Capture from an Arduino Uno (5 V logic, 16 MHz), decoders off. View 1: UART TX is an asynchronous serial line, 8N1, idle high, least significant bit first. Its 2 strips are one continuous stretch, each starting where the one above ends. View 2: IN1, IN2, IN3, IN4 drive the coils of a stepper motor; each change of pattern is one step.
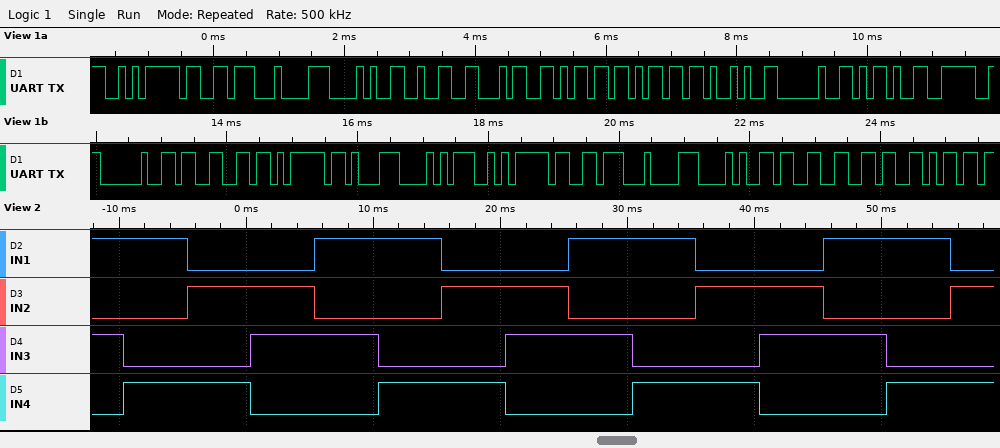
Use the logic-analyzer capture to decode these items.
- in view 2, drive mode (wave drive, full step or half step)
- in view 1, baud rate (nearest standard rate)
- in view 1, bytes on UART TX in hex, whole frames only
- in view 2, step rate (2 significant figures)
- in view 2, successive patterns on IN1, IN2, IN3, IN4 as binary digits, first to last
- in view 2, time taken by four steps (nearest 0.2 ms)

full step
9600 baud
EA B3 84 28 32 34 6D 6D 29 20 2D 3E 20 33 EB 8B A8 EA B3 84 28 33 36 6D
200 steps/s
1010 1001 0101 0110 1010 1001 0101 0110 1010 1001 0101 0110 1010 1001 0101
20.0 ms
